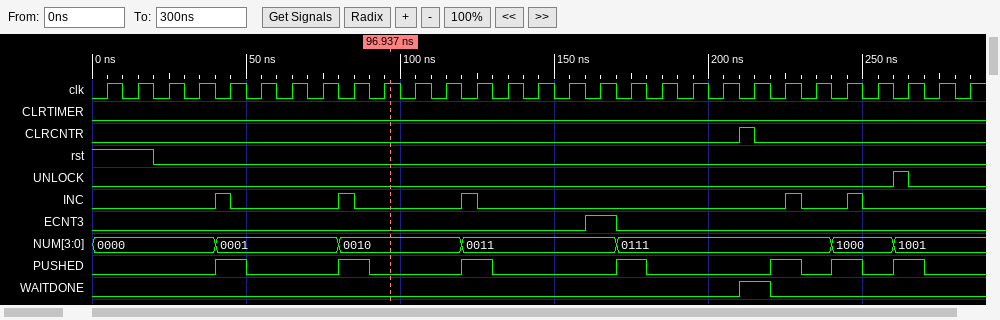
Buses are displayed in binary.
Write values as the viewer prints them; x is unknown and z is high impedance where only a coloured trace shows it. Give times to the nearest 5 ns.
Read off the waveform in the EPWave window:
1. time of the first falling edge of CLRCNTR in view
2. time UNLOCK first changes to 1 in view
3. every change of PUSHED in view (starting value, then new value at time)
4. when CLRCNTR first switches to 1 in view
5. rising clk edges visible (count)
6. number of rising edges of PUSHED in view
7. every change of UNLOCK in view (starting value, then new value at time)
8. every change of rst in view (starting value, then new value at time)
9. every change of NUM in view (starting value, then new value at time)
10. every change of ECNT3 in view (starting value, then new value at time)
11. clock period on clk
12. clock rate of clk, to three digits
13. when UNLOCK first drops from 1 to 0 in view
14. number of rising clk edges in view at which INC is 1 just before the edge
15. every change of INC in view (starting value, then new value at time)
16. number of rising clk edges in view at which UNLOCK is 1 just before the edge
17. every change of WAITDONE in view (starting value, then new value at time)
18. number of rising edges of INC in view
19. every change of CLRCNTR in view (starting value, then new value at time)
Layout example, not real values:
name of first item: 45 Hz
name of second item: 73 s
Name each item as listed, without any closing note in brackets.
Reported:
time of the first falling edge of CLRCNTR in view: 215 ns
time UNLOCK first changes to 1 in view: 260 ns
every change of PUSHED in view: 0, 1 at 40 ns, 0 at 50 ns, 1 at 80 ns, 0 at 90 ns, 1 at 120 ns, 0 at 130 ns, 1 at 170 ns, 0 at 180 ns, 1 at 220 ns, 0 at 230 ns, 1 at 240 ns, 0 at 250 ns, 1 at 260 ns, 0 at 270 ns
when CLRCNTR first switches to 1 in view: 210 ns
rising clk edges visible: 29
number of rising edges of PUSHED in view: 7
every change of UNLOCK in view: 0, 1 at 260 ns, 0 at 265 ns
every change of rst in view: 1, 0 at 20 ns
every change of NUM in view: 0000, 0001 at 40 ns, 0010 at 80 ns, 0011 at 120 ns, 0111 at 170 ns, 1000 at 240 ns, 1001 at 260 ns
every change of ECNT3 in view: 0, 1 at 160 ns, 0 at 170 ns
clock period on clk: 10 ns
clock rate of clk, to three digits: 100 MHz
when UNLOCK first drops from 1 to 0 in view: 265 ns
number of rising clk edges in view at which INC is 1 just before the edge: 3
every change of INC in view: 0, 1 at 40 ns, 0 at 45 ns, 1 at 80 ns, 0 at 85 ns, 1 at 120 ns, 0 at 125 ns, 1 at 225 ns, 0 at 230 ns, 1 at 245 ns, 0 at 250 ns
number of rising clk edges in view at which UNLOCK is 1 just before the edge: 1
every change of WAITDONE in view: 0, 1 at 210 ns, 0 at 220 ns
number of rising edges of INC in view: 5
every change of CLRCNTR in view: 0, 1 at 210 ns, 0 at 215 ns
